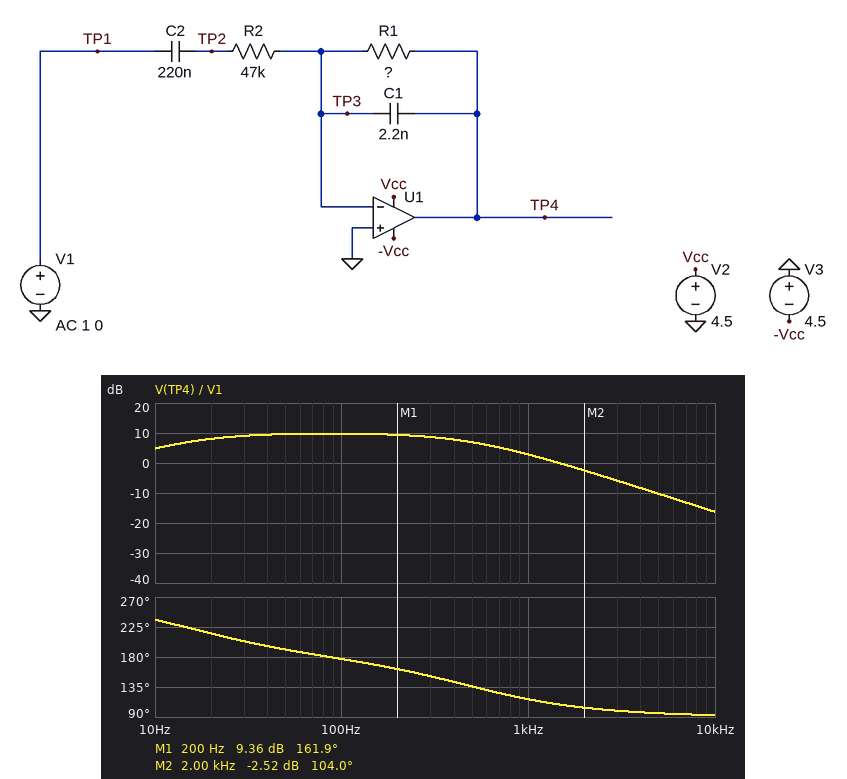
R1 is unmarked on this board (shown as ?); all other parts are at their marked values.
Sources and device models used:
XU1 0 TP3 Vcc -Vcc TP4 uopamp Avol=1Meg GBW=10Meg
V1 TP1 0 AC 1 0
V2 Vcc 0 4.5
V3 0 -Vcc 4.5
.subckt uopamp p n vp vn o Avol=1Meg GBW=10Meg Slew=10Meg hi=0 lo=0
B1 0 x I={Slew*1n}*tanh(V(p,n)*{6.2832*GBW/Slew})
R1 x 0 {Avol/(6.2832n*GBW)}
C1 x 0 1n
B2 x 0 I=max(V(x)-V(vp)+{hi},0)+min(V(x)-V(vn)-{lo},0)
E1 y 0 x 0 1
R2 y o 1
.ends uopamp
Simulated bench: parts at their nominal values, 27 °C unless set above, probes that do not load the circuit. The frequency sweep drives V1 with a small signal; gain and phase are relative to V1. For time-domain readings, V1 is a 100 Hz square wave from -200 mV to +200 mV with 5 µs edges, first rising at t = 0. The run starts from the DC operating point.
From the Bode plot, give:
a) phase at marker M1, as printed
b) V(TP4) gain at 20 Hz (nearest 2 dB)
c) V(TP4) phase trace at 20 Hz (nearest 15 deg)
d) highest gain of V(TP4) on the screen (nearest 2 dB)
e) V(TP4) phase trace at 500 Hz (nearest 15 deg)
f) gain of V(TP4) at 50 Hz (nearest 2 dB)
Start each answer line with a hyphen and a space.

- 161.9 deg
- 8 dB
- 210 deg
- 10 dB
- 135 deg
- 10 dB
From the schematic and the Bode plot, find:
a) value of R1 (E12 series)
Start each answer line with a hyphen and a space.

- 150 kΩ
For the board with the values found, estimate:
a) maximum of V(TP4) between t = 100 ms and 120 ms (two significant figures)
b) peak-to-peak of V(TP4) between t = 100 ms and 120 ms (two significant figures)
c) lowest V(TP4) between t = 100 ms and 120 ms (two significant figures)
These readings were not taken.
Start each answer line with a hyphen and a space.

- 690 mV
- 1.4 V
- -690 mV
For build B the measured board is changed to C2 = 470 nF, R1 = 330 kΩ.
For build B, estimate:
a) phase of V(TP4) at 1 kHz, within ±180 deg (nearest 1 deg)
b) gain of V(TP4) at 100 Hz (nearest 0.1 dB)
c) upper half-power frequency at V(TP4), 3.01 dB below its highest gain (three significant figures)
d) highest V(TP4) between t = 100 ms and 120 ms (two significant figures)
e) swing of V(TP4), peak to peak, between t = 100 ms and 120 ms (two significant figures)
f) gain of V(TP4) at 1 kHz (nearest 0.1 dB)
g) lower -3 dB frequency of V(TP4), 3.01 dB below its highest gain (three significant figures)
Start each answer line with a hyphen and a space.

- 103 deg
- 16.1 dB
- 233 Hz
- 1.4 V
- 2.7 V
- 3.5 dB
- 6.77 Hz
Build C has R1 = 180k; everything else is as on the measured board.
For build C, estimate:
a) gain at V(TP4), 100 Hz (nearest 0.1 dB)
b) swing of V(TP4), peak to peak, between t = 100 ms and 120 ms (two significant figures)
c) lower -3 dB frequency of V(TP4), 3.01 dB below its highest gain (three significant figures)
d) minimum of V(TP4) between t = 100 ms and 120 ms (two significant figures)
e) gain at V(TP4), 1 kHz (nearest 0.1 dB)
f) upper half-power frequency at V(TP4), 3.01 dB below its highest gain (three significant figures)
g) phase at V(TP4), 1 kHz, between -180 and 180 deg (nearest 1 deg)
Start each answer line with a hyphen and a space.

- 11.3 dB
- 1.6 V
- 14.3 Hz
- -820 mV
- 3.1 dB
- 432 Hz
- 113 deg
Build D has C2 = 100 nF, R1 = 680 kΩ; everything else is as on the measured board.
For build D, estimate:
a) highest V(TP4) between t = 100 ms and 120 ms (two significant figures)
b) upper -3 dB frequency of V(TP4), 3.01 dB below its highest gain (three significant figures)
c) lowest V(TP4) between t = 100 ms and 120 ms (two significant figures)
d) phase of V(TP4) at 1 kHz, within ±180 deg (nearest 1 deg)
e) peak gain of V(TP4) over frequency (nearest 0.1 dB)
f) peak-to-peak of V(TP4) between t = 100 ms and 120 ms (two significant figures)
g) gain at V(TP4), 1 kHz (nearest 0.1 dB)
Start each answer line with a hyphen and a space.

- 2.2 V
- 162 Hz
- -2.2 V
- 98 deg
- 20.8 dB
- 4.5 V
- 3.7 dB
